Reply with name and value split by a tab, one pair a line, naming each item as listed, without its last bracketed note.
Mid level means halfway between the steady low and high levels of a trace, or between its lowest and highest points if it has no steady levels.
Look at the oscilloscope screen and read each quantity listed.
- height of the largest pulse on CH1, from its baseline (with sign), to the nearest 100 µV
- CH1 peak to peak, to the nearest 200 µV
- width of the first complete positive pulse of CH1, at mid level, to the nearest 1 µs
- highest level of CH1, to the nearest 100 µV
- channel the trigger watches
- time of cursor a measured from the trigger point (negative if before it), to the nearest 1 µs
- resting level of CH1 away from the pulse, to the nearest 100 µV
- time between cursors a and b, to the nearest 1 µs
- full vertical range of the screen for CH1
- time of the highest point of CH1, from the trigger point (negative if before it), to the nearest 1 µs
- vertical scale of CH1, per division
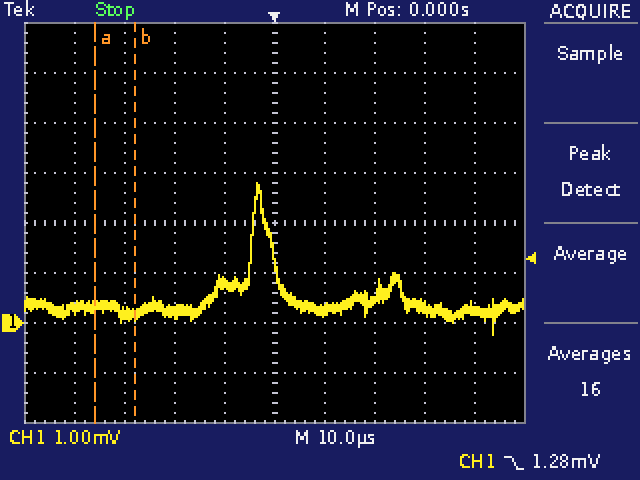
height of the largest pulse on CH1, from its baseline (with sign), to the nearest 100 µV	+2.5 mV
CH1 peak to peak, to the nearest 200 µV	3.0 mV
width of the first complete positive pulse of CH1, at mid level, to the nearest 1 µs	5 µs
highest level of CH1, to the nearest 100 µV	2.8 mV
channel the trigger watches	CH1
time of cursor a measured from the trigger point (negative if before it), to the nearest 1 µs	-36 µs
resting level of CH1 away from the pulse, to the nearest 100 µV	300 µV
time between cursors a and b, to the nearest 1 µs	8 µs
full vertical range of the screen for CH1	8 mV
time of the highest point of CH1, from the trigger point (negative if before it), to the nearest 1 µs	-3 µs
vertical scale of CH1, per division	1 mV
